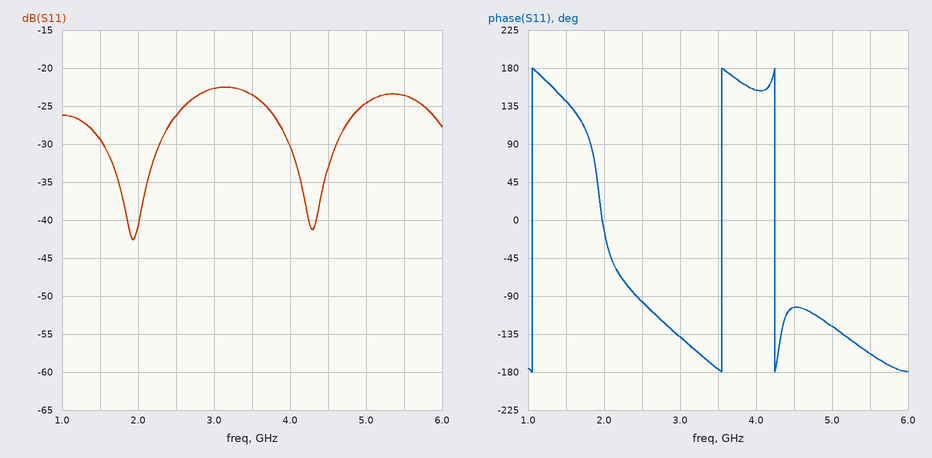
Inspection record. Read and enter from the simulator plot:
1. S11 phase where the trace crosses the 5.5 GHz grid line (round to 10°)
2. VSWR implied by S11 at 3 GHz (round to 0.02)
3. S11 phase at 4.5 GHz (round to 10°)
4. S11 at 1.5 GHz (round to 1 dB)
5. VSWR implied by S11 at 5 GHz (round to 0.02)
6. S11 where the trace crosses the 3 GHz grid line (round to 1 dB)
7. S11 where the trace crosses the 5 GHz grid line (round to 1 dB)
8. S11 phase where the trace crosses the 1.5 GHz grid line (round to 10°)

-160°
1.16
-100°
-29 dB
1.12
-23 dB
-25 dB
140°
